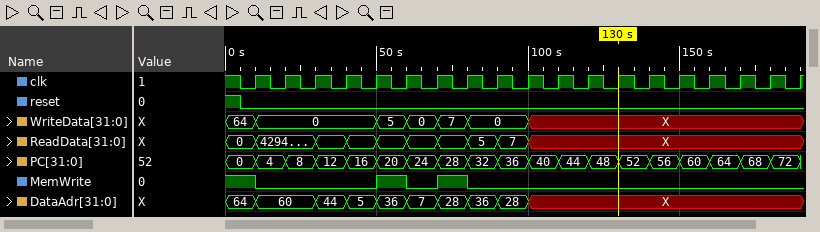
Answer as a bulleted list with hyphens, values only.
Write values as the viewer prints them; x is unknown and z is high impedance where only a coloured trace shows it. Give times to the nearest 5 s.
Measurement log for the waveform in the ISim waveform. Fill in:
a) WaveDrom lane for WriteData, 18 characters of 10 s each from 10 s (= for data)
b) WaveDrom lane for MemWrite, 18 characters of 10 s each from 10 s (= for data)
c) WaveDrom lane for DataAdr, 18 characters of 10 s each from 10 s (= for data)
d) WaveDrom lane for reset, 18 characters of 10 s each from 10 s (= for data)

- {name: 'WriteData', wave: '=...====.x........', data: '0 5 0 7 0'}
- {name: 'MemWrite', wave: '0...1010..........'}
- {name: 'DataAdr', wave: '=.=======x........', data: '60 44 5 36 7 28 36 28'}
- {name: 'reset', wave: '0.................'}
